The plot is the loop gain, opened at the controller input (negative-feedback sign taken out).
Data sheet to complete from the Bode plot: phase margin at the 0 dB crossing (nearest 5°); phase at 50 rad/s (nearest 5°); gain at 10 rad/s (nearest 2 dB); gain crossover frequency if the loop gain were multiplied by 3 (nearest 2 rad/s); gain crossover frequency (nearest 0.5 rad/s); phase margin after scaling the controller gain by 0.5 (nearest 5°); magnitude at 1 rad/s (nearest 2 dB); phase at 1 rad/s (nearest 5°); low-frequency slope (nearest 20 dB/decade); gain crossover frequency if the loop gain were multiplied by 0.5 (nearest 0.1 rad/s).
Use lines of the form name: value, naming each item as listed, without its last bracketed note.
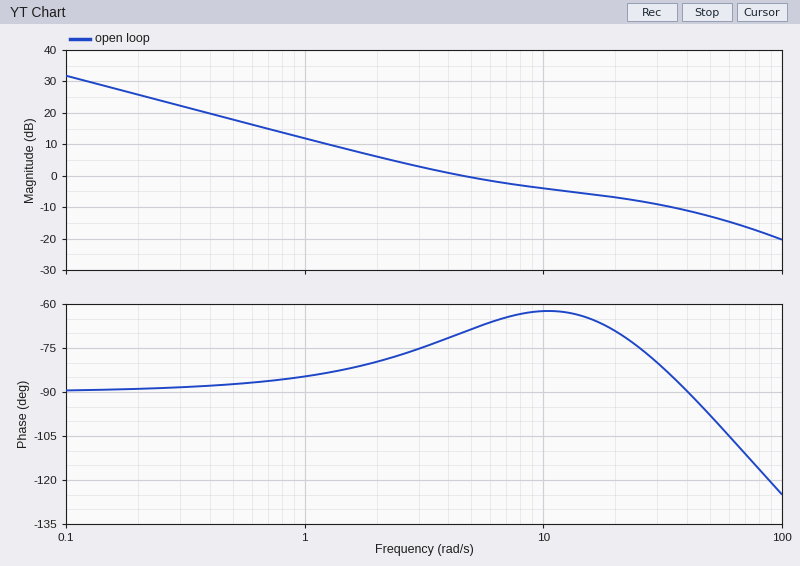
phase margin at the 0 dB crossing: 110°
phase at 50 rad/s: -100°
gain at 10 rad/s: -4 dB
gain crossover frequency if the loop gain were multiplied by 3: 32 rad/s
gain crossover frequency: 4.5 rad/s
phase margin after scaling the controller gain by 0.5: 100°
magnitude at 1 rad/s: 12 dB
phase at 1 rad/s: -85°
low-frequency slope: -20 dB/decade
gain crossover frequency if the loop gain were multiplied by 0.5: 2.0 rad/s
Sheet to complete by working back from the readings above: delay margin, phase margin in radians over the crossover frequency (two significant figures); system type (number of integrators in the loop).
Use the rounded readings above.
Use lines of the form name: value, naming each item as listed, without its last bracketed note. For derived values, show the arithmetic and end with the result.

delay margin, phase margin in radians over the crossover frequency: 110 × π / 180 / 4.5 = 0.43 s
system type: 1
